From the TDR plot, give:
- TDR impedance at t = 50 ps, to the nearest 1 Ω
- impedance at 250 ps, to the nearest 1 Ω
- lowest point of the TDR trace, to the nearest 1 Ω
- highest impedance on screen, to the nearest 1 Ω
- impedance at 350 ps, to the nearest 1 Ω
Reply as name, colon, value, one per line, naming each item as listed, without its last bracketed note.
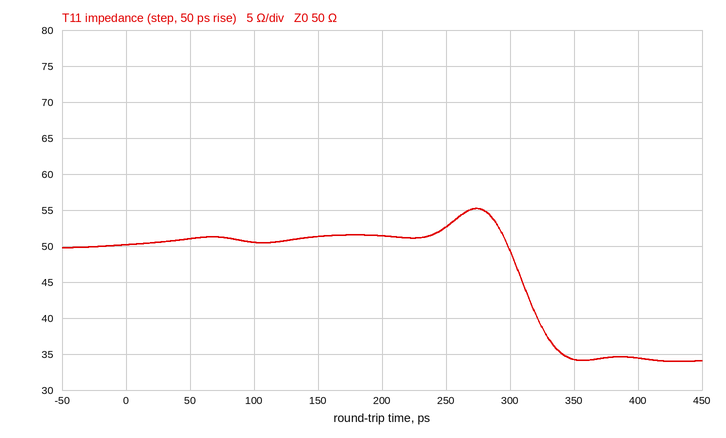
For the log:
TDR impedance at t = 50 ps, to the nearest 1 Ω: 51 Ω
impedance at 250 ps, to the nearest 1 Ω: 53 Ω
lowest point of the TDR trace, to the nearest 1 Ω: 34 Ω
highest impedance on screen, to the nearest 1 Ω: 55 Ω
impedance at 350 ps, to the nearest 1 Ω: 34 Ω
